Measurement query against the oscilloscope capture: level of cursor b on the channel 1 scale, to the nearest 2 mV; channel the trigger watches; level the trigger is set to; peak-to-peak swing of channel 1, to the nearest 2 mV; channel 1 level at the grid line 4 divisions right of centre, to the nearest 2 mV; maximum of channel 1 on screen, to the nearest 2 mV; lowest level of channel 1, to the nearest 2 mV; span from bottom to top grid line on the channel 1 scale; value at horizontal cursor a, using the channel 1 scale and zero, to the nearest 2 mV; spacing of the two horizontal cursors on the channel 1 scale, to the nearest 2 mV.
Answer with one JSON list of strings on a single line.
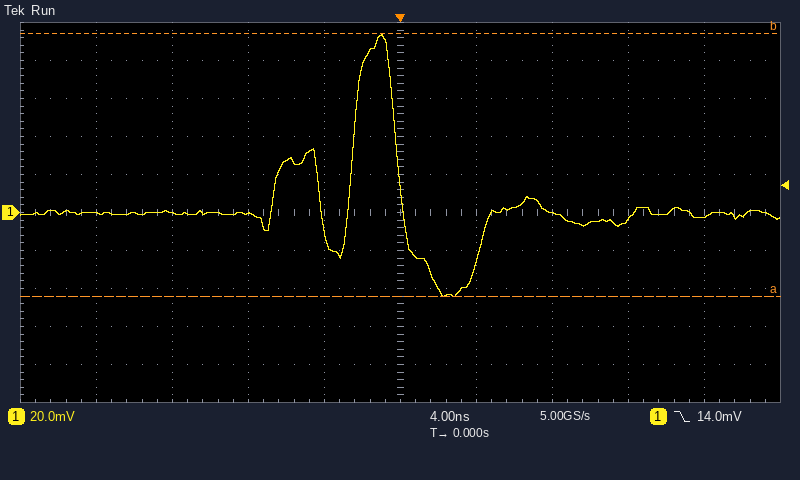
["94 mV", "channel 1", "14.0 mV", "138 mV", "-2 mV", "94 mV", "-44 mV", "200 mV", "-44 mV", "138 mV"]
